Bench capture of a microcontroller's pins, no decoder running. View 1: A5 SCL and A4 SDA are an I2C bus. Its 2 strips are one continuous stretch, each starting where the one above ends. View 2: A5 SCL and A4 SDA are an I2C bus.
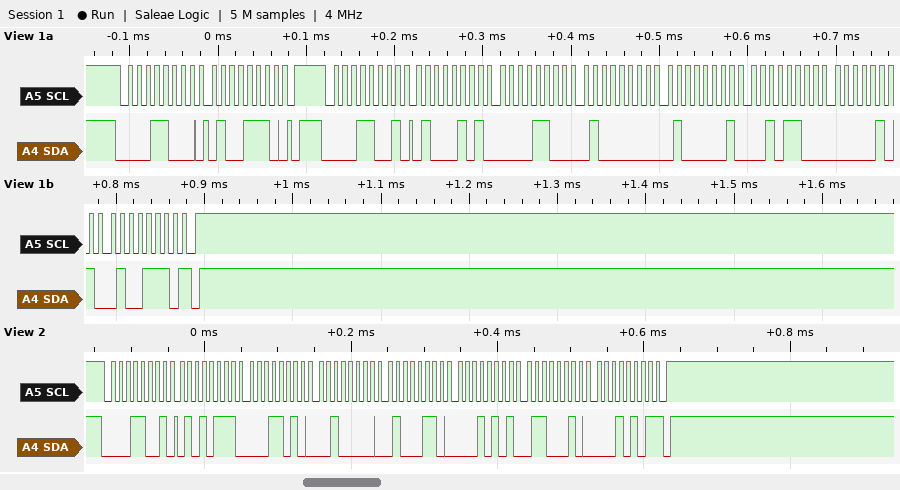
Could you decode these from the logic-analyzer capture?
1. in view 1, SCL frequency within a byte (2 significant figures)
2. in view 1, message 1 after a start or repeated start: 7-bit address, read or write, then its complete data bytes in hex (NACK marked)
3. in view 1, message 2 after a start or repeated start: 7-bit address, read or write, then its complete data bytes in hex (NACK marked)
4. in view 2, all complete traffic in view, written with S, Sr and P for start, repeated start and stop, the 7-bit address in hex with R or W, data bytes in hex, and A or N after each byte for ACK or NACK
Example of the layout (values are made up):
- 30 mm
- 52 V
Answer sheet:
- 100 kHz
- 0x0C write: 4E
- 0x0C read: 45 0C 40 41 2C 05 4E NACK
- S 0CR A 57 A 1A A 20 A 46 A 15 A 62 A 15 N P
